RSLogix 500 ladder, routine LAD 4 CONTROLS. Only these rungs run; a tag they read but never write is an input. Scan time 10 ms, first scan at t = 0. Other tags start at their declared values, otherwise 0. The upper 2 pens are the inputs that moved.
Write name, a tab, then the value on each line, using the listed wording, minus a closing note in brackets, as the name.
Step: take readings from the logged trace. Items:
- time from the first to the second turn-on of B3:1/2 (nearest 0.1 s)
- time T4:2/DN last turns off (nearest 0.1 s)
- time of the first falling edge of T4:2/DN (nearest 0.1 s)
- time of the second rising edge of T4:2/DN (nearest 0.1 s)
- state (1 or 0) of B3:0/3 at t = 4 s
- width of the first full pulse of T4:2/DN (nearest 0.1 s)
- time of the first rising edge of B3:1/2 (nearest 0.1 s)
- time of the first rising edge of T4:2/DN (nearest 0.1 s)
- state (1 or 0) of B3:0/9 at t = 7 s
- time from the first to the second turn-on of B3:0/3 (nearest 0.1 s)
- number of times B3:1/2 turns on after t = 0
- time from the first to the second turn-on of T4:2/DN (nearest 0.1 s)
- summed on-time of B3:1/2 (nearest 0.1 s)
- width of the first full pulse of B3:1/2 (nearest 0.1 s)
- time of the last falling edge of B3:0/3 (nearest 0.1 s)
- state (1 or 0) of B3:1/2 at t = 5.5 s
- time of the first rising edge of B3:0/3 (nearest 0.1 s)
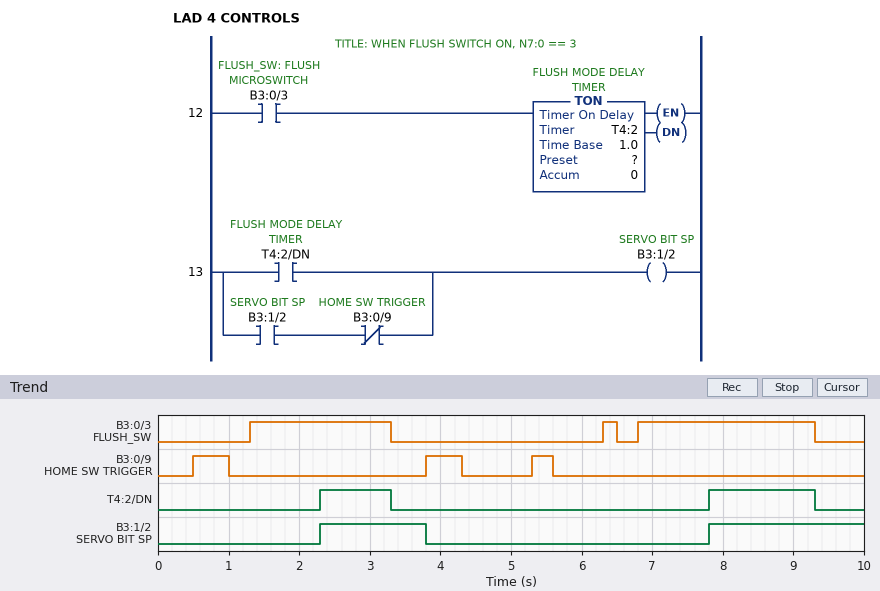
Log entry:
time from the first to the second turn-on of B3:1/2	5.5 s
time T4:2/DN last turns off	9.3 s
time of the first falling edge of T4:2/DN	3.3 s
time of the second rising edge of T4:2/DN	7.8 s
state (1 or 0) of B3:0/3 at t = 4 s	0
width of the first full pulse of T4:2/DN	1.0 s
time of the first rising edge of B3:1/2	2.3 s
time of the first rising edge of T4:2/DN	2.3 s
state (1 or 0) of B3:0/9 at t = 7 s	0
time from the first to the second turn-on of B3:0/3	5.0 s
number of times B3:1/2 turns on after t = 0	2
time from the first to the second turn-on of T4:2/DN	5.5 s
summed on-time of B3:1/2	3.7 s
width of the first full pulse of B3:1/2	1.5 s
time of the last falling edge of B3:0/3	9.3 s
state (1 or 0) of B3:1/2 at t = 5.5 s	0
time of the first rising edge of B3:0/3	1.3 s
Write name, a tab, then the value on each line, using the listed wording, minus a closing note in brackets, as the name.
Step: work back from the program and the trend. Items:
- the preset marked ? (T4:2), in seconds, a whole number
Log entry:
the preset marked ? (T4:2), in seconds, a whole number	1 s
